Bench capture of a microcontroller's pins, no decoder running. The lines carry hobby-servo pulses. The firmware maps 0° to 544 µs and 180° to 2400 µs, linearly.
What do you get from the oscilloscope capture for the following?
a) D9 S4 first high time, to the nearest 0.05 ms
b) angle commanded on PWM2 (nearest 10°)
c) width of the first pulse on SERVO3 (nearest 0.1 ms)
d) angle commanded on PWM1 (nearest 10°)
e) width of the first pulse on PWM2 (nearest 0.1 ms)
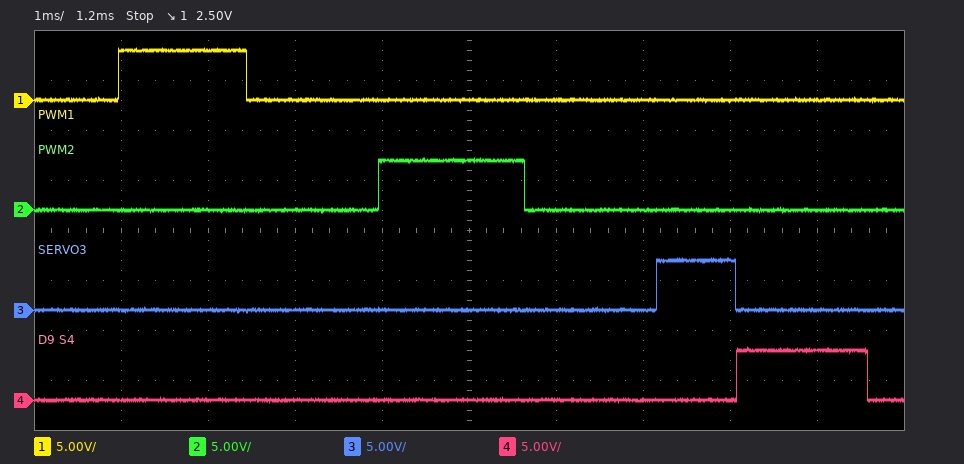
1.50 ms
110°
0.9 ms
90°
1.7 ms
